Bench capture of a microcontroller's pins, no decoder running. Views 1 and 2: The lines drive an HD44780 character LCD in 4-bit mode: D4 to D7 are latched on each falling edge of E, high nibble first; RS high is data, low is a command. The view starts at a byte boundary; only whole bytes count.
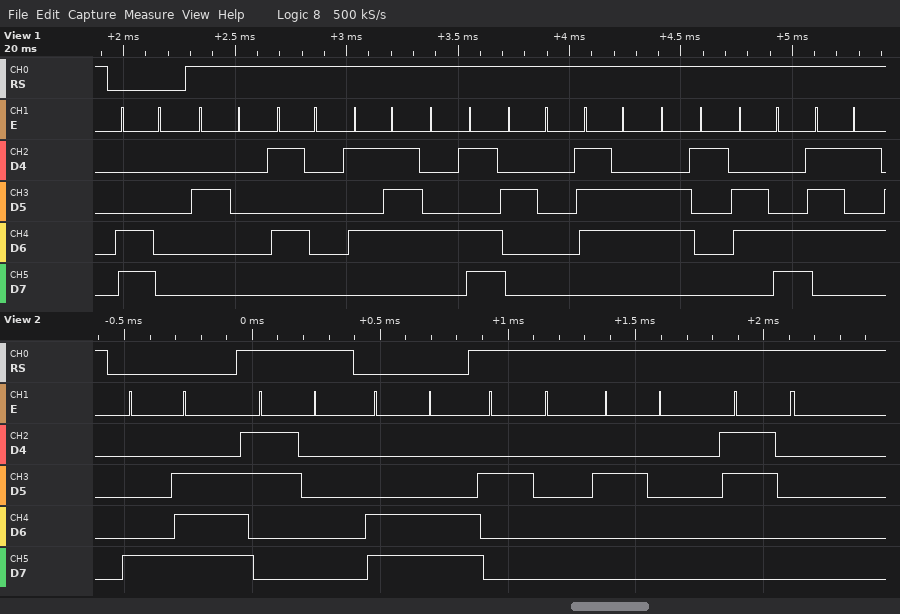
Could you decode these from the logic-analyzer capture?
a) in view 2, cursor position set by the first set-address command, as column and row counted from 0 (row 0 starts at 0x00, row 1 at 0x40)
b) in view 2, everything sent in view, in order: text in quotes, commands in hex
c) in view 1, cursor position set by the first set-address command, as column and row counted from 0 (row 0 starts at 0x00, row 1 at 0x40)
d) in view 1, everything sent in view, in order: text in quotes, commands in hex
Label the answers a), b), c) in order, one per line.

a) column 14, row 0
b) 0x8E "0" 0xCC "  0"
c) column 0, row 1
d) 0xC0 " PWM valu"
